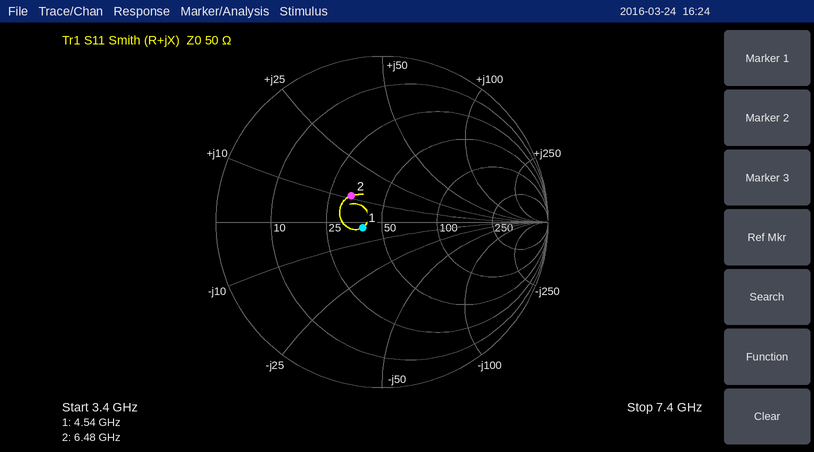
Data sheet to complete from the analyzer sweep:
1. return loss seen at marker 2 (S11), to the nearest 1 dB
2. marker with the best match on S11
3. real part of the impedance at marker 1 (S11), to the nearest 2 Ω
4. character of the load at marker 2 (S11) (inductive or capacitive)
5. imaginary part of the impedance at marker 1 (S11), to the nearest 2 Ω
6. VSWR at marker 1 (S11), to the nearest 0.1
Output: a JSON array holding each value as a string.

["12 dB", "marker 1", "40 Ω", "inductive", "-2 Ω", "1.3"]
